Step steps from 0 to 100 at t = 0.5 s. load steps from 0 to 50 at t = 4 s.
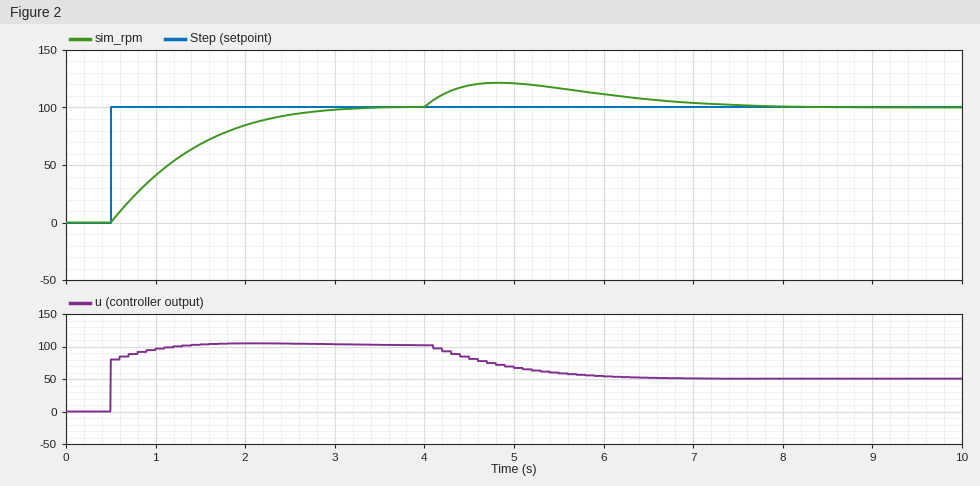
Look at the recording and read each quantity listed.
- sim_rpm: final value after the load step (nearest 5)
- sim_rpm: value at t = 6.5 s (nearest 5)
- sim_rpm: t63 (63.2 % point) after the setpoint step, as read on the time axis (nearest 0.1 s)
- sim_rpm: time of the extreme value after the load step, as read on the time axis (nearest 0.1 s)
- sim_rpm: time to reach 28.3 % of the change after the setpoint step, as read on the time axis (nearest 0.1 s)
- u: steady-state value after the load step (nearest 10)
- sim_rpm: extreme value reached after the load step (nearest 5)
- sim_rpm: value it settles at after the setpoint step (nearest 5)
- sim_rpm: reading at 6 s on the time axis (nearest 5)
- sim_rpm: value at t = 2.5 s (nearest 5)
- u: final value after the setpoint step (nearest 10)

100
105
1.4 s
4.8 s
0.8 s
50
120
100
110
95
100
